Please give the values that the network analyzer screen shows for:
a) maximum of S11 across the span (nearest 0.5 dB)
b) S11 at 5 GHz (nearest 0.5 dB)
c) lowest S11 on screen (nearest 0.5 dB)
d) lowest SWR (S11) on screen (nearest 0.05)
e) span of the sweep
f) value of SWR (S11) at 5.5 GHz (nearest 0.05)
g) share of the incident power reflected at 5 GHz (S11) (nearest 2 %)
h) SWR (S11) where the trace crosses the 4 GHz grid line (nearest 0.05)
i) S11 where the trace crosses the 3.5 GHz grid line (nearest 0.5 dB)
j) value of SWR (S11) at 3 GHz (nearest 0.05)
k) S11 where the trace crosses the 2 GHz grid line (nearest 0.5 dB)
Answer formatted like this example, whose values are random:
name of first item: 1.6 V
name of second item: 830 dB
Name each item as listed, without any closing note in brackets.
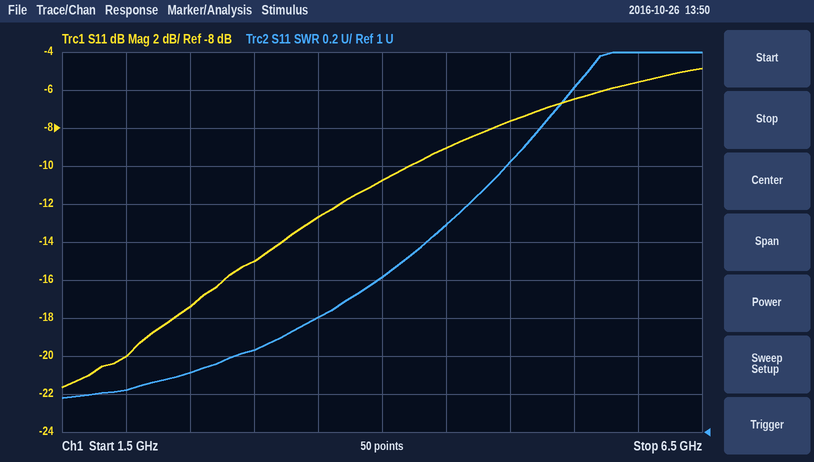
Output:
maximum of S11 across the span: -5.0 dB
S11 at 5 GHz: -7.5 dB
lowest S11 on screen: -21.5 dB
lowest SWR (S11) on screen: 1.20
span of the sweep: 5 GHz
value of SWR (S11) at 5.5 GHz: 2.80
share of the incident power reflected at 5 GHz (S11): 18 %
SWR (S11) where the trace crosses the 4 GHz grid line: 1.80
S11 where the trace crosses the 3.5 GHz grid line: -12.5 dB
value of SWR (S11) at 3 GHz: 1.45
S11 where the trace crosses the 2 GHz grid line: -20.0 dB
